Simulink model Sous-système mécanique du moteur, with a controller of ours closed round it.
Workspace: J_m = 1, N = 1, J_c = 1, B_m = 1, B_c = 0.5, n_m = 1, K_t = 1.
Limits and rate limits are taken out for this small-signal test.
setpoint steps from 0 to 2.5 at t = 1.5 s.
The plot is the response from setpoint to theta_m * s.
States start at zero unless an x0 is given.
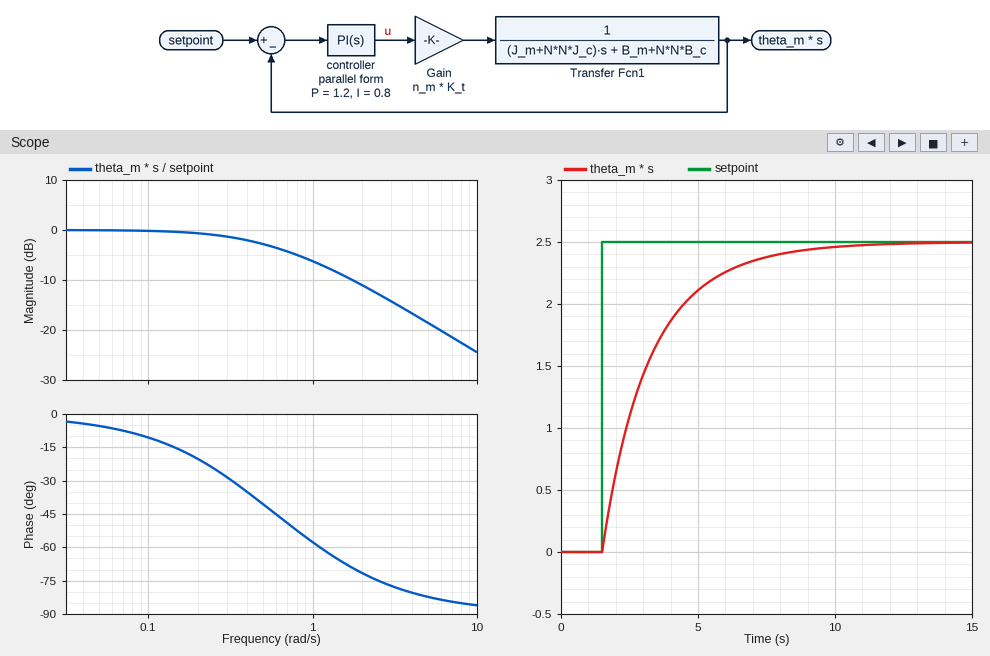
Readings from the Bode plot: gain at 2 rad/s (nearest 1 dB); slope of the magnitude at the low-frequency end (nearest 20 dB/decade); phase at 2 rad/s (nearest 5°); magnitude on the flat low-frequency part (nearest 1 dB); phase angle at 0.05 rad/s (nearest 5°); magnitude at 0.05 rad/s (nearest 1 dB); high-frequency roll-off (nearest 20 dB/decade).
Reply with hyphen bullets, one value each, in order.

- -11 dB
- 0 dB/decade
- -70°
- 0 dB
- -5°
- 0 dB
- -20 dB/decade
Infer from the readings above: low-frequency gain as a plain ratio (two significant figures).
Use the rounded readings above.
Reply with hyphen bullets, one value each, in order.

- 1.0
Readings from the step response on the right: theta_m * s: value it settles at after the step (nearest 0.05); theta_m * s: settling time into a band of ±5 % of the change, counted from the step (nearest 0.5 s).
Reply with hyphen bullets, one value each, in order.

- 2.50
- 6.0 s
